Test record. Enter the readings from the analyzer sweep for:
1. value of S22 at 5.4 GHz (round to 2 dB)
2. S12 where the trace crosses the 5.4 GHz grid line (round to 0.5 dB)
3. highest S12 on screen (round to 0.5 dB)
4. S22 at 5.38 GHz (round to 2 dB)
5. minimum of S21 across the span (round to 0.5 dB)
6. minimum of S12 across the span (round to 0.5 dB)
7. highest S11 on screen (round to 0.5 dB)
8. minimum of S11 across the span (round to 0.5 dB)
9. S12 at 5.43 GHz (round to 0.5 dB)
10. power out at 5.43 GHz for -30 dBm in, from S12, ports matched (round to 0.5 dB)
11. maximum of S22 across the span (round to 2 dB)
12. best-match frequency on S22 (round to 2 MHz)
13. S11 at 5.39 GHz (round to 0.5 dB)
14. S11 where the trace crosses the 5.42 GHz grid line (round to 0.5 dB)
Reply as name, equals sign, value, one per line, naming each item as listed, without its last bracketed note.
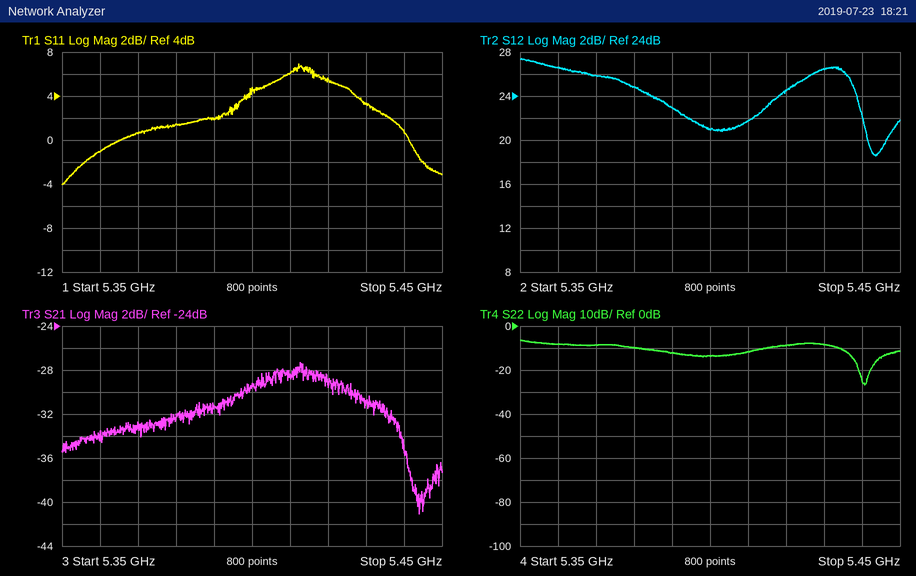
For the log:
value of S22 at 5.4 GHz = -14 dB
S12 where the trace crosses the 5.4 GHz grid line = 21.0 dB
highest S12 on screen = 27.5 dB
S22 at 5.38 GHz = -10 dB
minimum of S21 across the span = -41.0 dB
minimum of S12 across the span = 18.5 dB
highest S11 on screen = 7.0 dB
minimum of S11 across the span = -4.0 dB
S12 at 5.43 GHz = 26.5 dB
power out at 5.43 GHz for -30 dBm in, from S12, ports matched = -3.5 dBm
maximum of S22 across the span = -6 dB
best-match frequency on S22 = 5.440 GHz
S11 at 5.39 GHz = 2.0 dB
S11 where the trace crosses the 5.42 GHz grid line = 5.5 dB
